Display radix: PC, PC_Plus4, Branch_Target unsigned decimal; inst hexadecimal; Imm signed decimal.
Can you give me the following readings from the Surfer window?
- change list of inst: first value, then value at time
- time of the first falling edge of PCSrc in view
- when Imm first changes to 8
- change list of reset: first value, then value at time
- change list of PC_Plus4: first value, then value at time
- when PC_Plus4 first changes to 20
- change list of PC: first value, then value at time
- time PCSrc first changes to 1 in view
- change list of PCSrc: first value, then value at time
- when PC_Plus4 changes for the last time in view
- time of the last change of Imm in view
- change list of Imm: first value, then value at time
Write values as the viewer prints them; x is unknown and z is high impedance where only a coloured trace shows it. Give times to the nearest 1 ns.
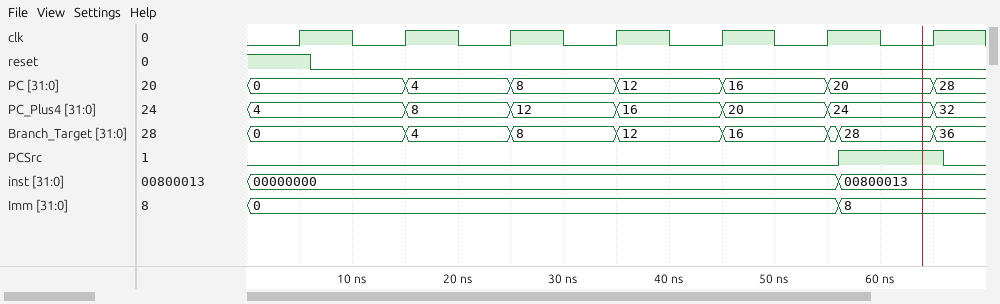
00000000, 00800013 at 56 ns
66 ns
56 ns
1, 0 at 6 ns
4, 8 at 15 ns, 12 at 25 ns, 16 at 35 ns, 20 at 45 ns, 24 at 55 ns, 32 at 65 ns
45 ns
0, 4 at 15 ns, 8 at 25 ns, 12 at 35 ns, 16 at 45 ns, 20 at 55 ns, 28 at 65 ns
56 ns
0, 1 at 56 ns, 0 at 66 ns
65 ns
56 ns
0, 8 at 56 ns
